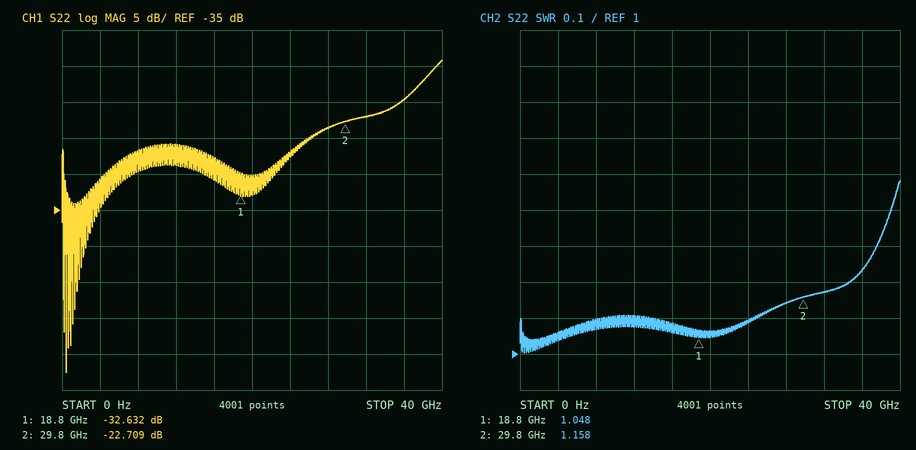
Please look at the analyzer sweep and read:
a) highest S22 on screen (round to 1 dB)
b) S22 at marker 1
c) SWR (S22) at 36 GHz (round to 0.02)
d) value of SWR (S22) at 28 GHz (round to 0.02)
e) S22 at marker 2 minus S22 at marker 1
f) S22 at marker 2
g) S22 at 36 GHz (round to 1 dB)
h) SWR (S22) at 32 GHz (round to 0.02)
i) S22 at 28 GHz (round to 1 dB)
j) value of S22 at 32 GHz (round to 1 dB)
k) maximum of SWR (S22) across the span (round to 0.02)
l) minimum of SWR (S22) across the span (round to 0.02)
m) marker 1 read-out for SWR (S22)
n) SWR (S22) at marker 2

-14 dB
-32.632 dB
1.24
1.14
9.923 dB
-22.709 dB
-20 dB
1.18
-24 dB
-22 dB
1.48
1.00
1.048
1.158
